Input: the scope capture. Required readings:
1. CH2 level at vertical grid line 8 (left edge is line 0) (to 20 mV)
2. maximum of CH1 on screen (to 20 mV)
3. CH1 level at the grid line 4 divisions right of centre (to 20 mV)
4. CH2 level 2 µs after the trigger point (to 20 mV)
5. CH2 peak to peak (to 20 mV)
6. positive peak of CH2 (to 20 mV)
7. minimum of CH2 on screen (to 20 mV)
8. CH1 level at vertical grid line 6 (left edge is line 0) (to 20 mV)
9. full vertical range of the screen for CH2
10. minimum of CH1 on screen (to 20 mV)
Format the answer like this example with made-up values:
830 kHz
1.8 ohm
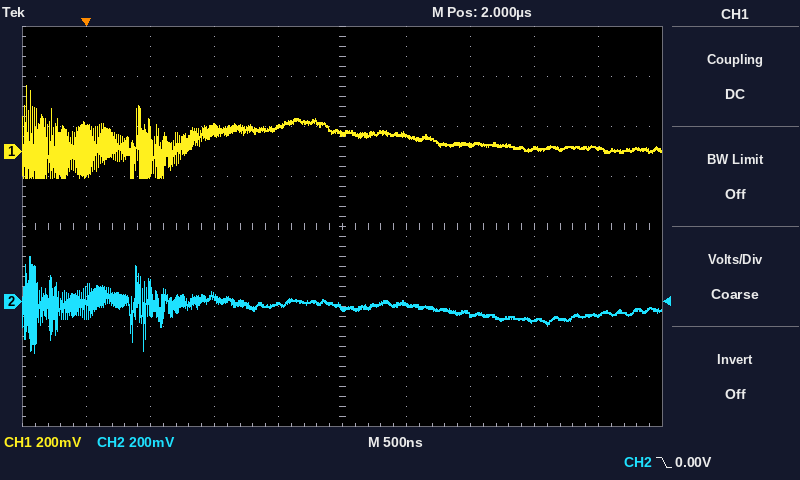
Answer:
-80 mV
260 mV
20 mV
-20 mV
380 mV
180 mV
-200 mV
60 mV
1.6 V
-100 mV
